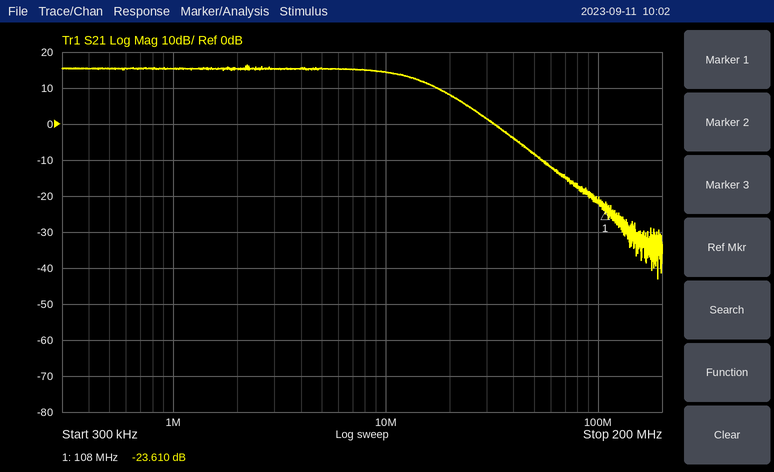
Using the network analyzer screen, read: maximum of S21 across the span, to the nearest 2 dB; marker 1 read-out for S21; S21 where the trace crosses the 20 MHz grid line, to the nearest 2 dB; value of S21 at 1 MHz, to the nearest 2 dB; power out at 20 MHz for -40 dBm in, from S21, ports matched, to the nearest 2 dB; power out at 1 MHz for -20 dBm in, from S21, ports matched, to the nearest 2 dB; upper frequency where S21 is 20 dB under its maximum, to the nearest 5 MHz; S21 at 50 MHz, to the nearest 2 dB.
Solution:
16 dB
-23.610 dB
8 dB
16 dB
-32 dBm
-4 dBm
40 MHz
-8 dB
